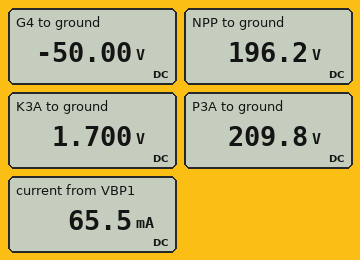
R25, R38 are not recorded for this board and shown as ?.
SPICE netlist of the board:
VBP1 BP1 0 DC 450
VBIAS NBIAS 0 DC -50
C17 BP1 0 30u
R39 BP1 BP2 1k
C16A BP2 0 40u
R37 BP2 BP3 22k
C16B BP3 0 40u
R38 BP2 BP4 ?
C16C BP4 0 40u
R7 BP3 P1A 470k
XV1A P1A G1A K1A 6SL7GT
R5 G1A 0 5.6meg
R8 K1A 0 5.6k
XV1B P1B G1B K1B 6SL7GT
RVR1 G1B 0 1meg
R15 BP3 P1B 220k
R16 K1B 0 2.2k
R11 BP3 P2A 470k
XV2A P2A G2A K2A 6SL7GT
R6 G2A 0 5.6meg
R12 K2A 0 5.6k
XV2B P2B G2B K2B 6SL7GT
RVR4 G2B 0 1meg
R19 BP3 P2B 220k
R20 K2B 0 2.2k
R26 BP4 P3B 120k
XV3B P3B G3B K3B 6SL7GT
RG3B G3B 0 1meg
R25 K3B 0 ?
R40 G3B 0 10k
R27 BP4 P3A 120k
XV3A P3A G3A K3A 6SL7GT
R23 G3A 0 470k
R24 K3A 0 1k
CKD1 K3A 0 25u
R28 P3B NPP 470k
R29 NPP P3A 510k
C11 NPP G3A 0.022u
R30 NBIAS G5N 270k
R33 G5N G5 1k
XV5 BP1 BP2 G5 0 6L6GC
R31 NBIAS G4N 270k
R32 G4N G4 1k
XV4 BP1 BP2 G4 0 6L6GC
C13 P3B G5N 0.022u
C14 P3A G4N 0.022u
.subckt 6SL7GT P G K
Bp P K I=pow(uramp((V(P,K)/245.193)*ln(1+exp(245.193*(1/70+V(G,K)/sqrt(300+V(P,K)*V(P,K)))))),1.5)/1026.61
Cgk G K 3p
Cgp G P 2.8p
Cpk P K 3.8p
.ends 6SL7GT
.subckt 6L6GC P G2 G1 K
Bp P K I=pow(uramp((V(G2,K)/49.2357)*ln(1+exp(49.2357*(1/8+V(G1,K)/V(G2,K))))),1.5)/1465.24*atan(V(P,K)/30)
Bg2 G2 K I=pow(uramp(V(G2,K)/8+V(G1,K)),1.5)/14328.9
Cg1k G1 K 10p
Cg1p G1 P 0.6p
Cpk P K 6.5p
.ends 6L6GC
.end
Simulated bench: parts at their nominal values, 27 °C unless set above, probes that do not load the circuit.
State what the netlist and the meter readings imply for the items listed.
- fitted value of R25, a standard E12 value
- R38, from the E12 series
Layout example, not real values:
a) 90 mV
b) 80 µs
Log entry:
a) 560 Ω
b) 6.8 kΩ
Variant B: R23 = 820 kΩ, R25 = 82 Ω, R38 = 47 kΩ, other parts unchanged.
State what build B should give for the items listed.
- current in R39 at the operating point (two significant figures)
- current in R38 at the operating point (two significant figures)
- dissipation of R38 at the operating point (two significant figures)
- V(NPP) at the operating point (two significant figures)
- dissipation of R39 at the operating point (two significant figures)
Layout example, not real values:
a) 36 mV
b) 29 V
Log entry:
a) 7.3 mA
b) 2.9 mA
c) 390 mW
d) 130 V
e) 53 mW
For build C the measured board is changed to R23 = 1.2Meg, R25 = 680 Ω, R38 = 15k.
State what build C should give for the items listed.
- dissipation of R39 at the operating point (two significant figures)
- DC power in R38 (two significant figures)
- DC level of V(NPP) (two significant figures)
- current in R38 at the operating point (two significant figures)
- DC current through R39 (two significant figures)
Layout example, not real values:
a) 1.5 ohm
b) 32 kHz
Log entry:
a) 59 mW
b) 170 mW
c) 190 V
d) 3.4 mA
e) 7.7 mA
